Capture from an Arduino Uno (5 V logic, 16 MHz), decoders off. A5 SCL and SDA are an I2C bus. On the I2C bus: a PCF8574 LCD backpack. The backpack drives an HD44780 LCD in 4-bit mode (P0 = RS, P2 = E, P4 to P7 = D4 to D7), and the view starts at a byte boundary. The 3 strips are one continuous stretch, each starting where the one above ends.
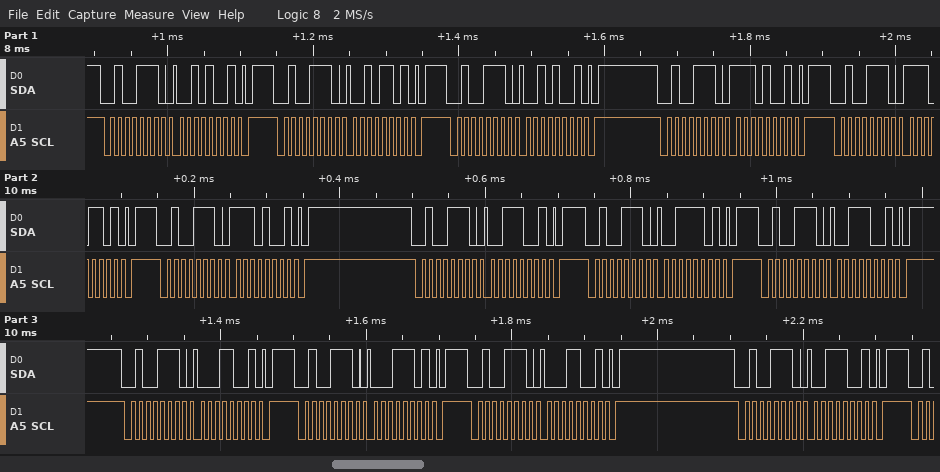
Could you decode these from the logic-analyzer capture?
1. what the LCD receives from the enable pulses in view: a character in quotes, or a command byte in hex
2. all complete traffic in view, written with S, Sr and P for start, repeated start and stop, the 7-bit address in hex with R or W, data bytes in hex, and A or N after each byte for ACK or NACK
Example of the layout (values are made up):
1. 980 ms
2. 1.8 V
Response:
1. '.' '1'
2. S 27W A 29 A P S 27W A 2D A P S 27W A 29 A P S 27W A E9 A P S 27W A ED A P S 27W A E9 A P S 27W A 39 A P S 27W A 3D A P S 27W A 39 A P S 27W A 19 A P S 27W A 1D A P S 27W A 19 A P S 27W A 39 A P
